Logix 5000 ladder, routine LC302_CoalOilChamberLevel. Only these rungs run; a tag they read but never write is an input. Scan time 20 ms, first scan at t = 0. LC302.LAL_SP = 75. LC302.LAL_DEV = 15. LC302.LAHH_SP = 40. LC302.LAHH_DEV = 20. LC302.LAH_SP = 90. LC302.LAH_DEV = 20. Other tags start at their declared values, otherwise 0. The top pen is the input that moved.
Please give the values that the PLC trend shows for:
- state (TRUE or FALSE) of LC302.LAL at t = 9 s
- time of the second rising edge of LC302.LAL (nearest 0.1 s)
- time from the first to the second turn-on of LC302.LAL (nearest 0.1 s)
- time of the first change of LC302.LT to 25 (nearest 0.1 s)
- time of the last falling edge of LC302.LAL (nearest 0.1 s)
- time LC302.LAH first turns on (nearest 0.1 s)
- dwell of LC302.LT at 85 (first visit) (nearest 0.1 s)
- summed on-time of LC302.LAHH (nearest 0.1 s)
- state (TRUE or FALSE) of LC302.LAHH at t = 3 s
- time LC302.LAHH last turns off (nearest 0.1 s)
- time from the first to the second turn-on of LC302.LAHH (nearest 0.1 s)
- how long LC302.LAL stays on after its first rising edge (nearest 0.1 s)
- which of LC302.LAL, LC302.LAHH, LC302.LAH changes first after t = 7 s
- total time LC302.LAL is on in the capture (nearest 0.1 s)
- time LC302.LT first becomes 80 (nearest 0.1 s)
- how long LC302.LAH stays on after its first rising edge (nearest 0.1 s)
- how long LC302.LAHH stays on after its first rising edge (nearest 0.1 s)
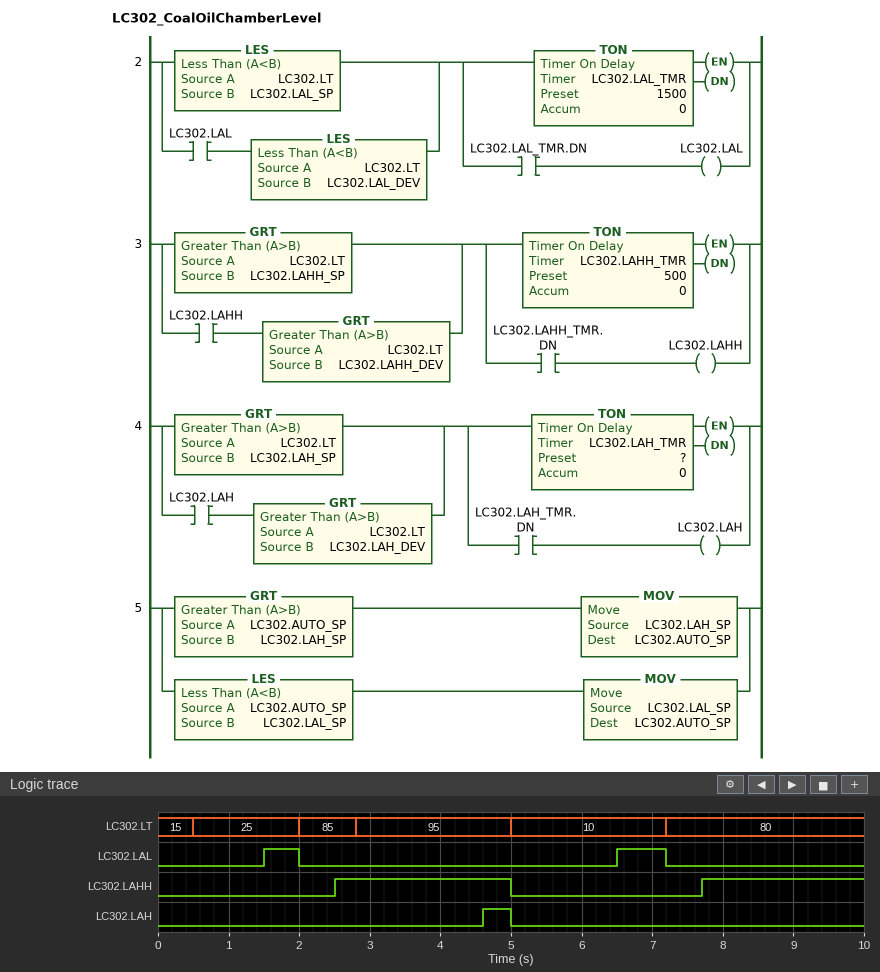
FALSE
6.5 s
5.0 s
0.5 s
7.2 s
4.6 s
0.8 s
4.8 s
TRUE
5.0 s
5.2 s
0.5 s
LC302.LAL
1.2 s
7.2 s
0.4 s
2.5 s
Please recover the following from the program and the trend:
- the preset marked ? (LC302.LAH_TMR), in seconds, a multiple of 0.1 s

1.8 s
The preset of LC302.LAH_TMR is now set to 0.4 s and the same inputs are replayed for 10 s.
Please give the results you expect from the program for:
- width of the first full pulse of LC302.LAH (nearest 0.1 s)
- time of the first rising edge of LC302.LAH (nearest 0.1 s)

1.8 s
3.2 s
